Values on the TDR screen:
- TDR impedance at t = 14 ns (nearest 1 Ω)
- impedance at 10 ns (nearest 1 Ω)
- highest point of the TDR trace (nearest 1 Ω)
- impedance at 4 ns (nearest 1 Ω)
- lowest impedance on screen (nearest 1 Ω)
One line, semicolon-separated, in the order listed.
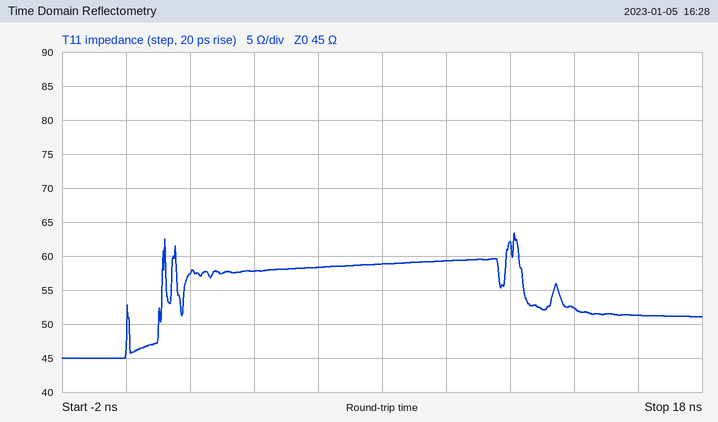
52 Ω; 59 Ω; 63 Ω; 58 Ω; 45 Ω
